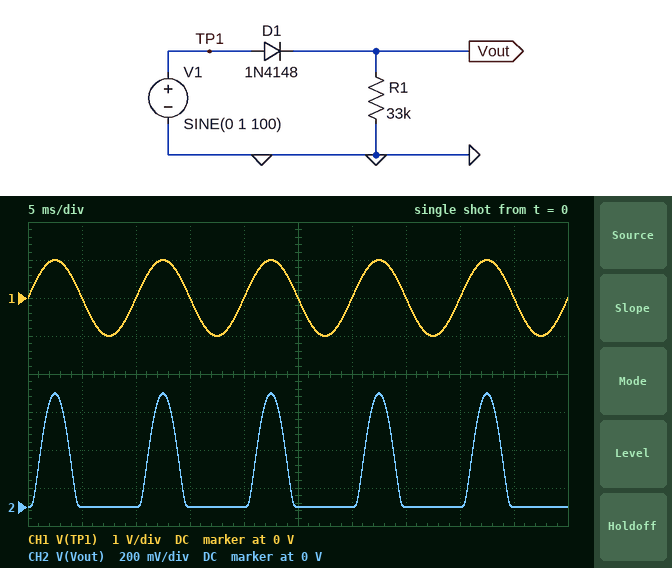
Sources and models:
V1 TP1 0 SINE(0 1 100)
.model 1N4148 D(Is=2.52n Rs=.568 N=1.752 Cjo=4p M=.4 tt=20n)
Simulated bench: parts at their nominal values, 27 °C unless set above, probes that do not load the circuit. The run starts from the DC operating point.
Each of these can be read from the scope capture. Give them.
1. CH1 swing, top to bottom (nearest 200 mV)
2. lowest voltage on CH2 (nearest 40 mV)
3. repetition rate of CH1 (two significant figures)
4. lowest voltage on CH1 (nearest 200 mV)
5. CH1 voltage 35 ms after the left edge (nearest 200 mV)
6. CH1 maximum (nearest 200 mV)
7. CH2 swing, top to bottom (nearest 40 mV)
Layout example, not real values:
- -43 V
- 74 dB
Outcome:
- 2.0 V
- 0 V
- 100 Hz
- -1.0 V
- 0 V
- 1.0 V
- 600 mV
